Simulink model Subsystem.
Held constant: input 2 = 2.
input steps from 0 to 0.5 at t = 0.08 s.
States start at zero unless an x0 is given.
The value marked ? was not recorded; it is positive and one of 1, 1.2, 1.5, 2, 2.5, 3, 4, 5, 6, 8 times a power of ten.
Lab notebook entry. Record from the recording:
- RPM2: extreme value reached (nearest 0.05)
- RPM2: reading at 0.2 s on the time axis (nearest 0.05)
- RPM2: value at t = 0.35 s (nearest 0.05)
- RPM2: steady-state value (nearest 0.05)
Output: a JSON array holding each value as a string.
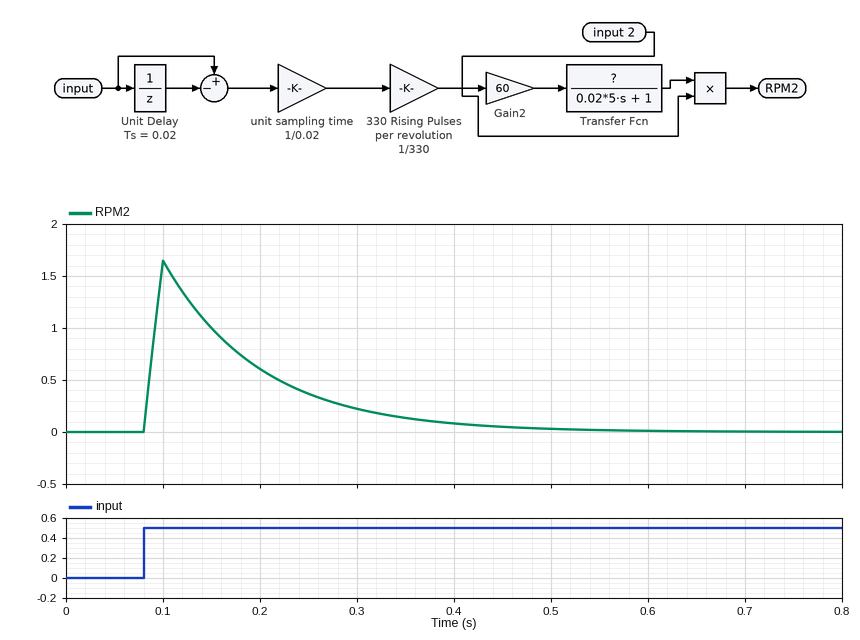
["1.65", "0.60", "0.15", "0.00"]
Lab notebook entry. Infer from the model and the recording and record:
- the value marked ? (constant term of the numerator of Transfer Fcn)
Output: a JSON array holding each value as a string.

["1"]
